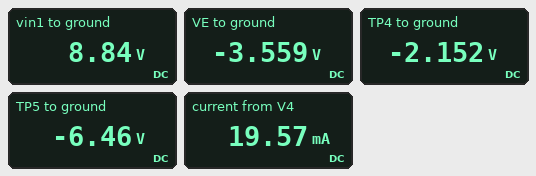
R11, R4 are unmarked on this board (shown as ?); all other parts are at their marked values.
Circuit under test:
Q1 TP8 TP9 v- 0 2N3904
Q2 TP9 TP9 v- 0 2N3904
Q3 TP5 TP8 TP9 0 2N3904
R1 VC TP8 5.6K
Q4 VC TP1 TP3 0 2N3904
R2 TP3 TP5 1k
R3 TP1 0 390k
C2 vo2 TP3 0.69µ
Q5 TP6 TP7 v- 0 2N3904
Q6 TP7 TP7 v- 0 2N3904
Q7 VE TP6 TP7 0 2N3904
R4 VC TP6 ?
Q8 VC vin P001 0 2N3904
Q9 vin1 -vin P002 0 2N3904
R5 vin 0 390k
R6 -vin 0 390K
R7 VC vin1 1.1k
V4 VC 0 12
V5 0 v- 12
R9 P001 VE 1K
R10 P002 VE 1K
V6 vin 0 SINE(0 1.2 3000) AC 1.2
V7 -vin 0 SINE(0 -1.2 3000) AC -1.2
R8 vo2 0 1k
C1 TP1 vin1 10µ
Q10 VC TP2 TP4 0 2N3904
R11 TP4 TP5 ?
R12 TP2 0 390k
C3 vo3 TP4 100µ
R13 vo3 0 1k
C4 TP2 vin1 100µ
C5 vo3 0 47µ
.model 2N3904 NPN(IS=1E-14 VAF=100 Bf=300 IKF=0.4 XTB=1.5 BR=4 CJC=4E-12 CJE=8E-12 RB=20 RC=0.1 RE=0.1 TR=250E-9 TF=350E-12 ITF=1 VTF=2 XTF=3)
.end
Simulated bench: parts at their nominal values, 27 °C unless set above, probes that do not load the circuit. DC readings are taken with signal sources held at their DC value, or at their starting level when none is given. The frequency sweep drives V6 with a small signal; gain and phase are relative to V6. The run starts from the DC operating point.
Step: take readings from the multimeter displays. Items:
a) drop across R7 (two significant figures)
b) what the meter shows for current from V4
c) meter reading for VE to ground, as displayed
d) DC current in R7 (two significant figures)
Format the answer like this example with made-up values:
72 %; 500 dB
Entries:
3.2 V; 19.57 mA; -3.559 V; 2.9 mA
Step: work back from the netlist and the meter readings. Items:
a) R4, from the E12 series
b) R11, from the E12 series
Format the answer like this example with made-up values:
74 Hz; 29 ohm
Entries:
3.9 kΩ; 3.3 kΩ
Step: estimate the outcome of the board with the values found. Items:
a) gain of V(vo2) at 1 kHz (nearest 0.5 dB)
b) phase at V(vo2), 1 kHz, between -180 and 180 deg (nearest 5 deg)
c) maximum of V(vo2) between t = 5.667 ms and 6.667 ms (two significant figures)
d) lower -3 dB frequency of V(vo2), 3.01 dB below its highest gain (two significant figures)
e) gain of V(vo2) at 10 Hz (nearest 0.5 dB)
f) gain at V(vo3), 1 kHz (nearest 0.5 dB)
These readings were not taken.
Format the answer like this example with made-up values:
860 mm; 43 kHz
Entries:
0 dB; 10 deg; 1.2 V; 190 Hz; -26.0 dB; -15.5 dB
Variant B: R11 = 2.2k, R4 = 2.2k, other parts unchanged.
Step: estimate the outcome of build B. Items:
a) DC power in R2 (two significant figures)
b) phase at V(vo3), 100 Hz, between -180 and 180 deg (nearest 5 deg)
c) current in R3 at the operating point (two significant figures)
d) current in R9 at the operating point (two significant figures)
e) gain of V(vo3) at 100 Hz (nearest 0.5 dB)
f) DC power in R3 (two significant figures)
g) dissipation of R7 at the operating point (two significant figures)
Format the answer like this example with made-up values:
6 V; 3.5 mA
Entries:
6.0 mW; -20 deg; 7.1 µA; 5.1 mA; -2.5 dB; 20 µW; 28 mW
